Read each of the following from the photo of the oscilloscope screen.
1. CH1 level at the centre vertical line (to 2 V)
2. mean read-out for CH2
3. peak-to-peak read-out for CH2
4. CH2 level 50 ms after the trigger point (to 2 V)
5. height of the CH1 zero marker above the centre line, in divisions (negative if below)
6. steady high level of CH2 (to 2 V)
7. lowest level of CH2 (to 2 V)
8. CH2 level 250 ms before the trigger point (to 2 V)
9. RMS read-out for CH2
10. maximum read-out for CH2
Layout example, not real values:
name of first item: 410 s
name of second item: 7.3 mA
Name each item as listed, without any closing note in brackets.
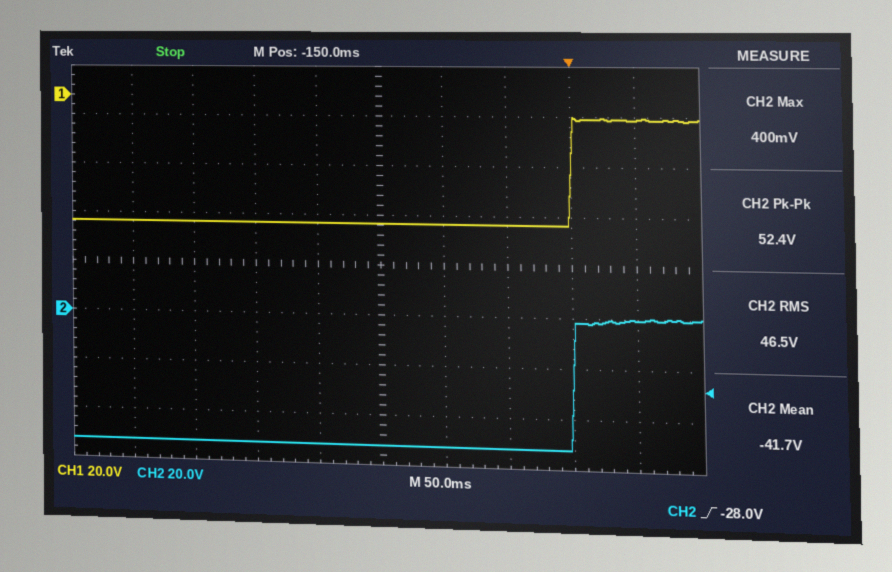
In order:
CH1 level at the centre vertical line: -52 V
mean read-out for CH2: -41.7 V
peak-to-peak read-out for CH2: 52.4 V
CH2 level 50 ms after the trigger point: 0 V
height of the CH1 zero marker above the centre line, in divisions: +3.4 div
steady high level of CH2: 0 V
lowest level of CH2: -52 V
CH2 level 250 ms before the trigger point: -52 V
RMS read-out for CH2: 46.5 V
maximum read-out for CH2: 400 mV
